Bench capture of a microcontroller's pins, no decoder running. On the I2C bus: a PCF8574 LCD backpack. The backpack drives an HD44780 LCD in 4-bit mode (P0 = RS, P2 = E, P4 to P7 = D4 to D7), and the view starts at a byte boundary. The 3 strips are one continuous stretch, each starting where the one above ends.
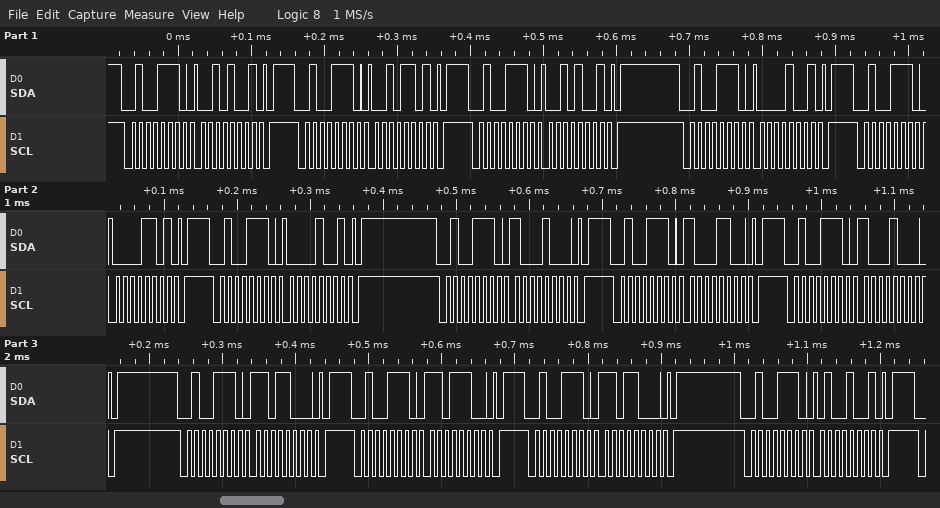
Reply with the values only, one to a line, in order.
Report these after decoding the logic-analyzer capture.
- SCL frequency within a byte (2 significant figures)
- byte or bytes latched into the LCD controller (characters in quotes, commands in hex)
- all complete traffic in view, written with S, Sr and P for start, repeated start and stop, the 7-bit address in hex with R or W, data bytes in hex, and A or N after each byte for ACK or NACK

100 kHz
' ' 0x8D
S 27W A 29 A P S 27W A 2D A P S 27W A 29 A P S 27W A 09 A P S 27W A 0D A P S 27W A 09 A P S 27W A 88 A P S 27W A 8C A P S 27W A 88 A P S 27W A D8 A P S 27W A DC A P S 27W A D8 A P S 27W A 49 A P
